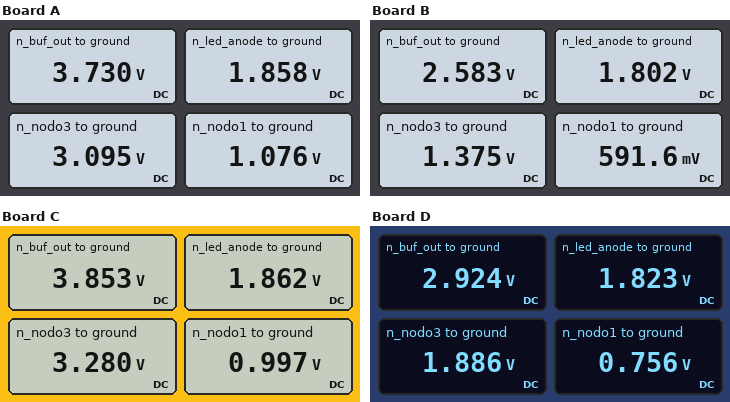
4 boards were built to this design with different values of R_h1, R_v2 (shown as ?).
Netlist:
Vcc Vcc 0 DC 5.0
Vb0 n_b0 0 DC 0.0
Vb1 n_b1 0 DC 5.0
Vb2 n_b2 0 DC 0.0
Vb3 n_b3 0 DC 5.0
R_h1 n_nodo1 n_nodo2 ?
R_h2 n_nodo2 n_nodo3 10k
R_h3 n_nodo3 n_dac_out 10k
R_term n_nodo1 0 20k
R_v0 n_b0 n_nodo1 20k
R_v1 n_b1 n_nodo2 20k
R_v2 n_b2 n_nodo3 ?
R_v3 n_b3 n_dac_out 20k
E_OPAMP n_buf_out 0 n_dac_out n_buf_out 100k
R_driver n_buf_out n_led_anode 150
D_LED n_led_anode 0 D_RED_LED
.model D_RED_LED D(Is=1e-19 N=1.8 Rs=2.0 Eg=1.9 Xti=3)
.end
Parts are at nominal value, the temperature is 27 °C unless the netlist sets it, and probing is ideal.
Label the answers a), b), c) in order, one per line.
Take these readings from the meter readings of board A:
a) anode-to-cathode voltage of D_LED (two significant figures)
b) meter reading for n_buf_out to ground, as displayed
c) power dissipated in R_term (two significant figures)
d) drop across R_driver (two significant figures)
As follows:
a) 1.9 V
b) 3.730 V
c) 58 µW
d) 1.9 V
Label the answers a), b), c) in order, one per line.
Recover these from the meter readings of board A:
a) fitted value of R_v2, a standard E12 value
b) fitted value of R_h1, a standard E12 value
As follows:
a) 56 kΩ
b) 18 kΩ
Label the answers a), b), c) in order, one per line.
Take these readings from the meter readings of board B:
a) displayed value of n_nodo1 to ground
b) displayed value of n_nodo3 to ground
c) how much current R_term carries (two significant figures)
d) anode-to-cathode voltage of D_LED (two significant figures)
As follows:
a) 591.6 mV
b) 1.375 V
c) 30 µA
d) 1.8 V
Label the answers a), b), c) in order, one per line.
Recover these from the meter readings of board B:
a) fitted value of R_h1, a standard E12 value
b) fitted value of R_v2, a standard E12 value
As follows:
a) 27 kΩ
b) 6.8 kΩ
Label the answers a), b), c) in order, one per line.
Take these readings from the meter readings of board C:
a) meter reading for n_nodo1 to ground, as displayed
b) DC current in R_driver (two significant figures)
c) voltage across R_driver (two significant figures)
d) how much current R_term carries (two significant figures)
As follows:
a) 0.997 V
b) 13 mA
c) 2.0 V
d) 50 µA
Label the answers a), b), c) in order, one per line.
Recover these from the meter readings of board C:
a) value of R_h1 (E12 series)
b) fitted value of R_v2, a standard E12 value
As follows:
a) 22 kΩ
b) 68 kΩ
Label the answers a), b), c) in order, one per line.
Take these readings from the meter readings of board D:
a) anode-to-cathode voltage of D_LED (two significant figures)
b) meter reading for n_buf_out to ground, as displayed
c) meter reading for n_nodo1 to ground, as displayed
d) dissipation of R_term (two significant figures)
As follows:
a) 1.8 V
b) 2.924 V
c) 0.756 V
d) 29 µW
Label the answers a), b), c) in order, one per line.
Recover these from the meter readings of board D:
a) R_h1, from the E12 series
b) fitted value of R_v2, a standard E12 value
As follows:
a) 22 kΩ
b) 12 kΩ
